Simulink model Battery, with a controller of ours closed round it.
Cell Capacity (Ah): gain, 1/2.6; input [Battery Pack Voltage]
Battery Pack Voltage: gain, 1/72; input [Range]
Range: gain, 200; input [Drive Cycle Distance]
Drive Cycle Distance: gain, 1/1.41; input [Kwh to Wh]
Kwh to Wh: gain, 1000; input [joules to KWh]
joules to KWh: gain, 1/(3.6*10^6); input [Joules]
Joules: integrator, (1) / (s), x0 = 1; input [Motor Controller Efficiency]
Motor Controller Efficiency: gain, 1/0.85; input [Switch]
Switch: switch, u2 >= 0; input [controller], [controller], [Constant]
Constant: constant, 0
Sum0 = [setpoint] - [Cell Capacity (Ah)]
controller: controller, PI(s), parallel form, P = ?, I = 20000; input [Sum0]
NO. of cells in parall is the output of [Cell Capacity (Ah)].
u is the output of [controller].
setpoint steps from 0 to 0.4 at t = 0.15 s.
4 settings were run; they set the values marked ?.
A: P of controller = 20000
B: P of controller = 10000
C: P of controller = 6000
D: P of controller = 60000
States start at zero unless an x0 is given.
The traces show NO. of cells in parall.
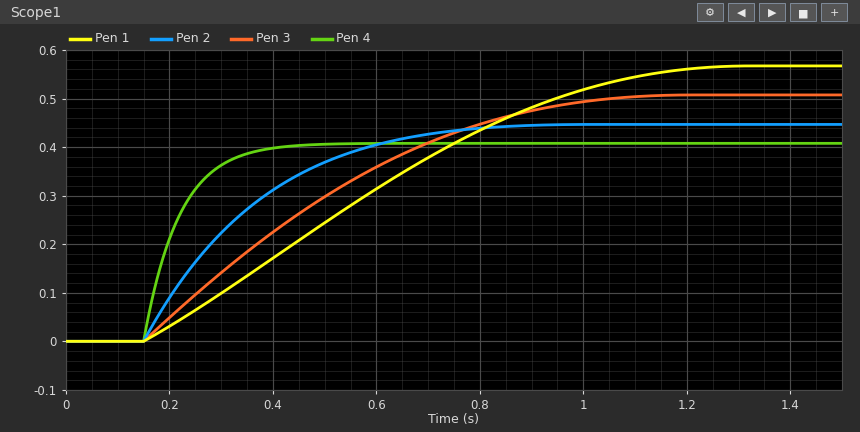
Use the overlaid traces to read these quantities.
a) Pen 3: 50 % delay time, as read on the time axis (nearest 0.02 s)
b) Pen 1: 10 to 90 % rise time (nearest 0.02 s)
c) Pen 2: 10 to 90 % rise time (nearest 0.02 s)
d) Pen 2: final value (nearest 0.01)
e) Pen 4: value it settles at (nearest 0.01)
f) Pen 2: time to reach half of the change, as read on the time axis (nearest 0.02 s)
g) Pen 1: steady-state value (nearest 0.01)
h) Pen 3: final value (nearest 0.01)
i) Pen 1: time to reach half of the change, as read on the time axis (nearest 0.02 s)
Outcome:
0.44 s
0.74 s
0.42 s
0.45
0.41
0.30 s
0.57
0.51
0.56 s
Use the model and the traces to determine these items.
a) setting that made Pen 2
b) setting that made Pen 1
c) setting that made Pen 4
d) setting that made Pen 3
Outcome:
A
C
D
B
